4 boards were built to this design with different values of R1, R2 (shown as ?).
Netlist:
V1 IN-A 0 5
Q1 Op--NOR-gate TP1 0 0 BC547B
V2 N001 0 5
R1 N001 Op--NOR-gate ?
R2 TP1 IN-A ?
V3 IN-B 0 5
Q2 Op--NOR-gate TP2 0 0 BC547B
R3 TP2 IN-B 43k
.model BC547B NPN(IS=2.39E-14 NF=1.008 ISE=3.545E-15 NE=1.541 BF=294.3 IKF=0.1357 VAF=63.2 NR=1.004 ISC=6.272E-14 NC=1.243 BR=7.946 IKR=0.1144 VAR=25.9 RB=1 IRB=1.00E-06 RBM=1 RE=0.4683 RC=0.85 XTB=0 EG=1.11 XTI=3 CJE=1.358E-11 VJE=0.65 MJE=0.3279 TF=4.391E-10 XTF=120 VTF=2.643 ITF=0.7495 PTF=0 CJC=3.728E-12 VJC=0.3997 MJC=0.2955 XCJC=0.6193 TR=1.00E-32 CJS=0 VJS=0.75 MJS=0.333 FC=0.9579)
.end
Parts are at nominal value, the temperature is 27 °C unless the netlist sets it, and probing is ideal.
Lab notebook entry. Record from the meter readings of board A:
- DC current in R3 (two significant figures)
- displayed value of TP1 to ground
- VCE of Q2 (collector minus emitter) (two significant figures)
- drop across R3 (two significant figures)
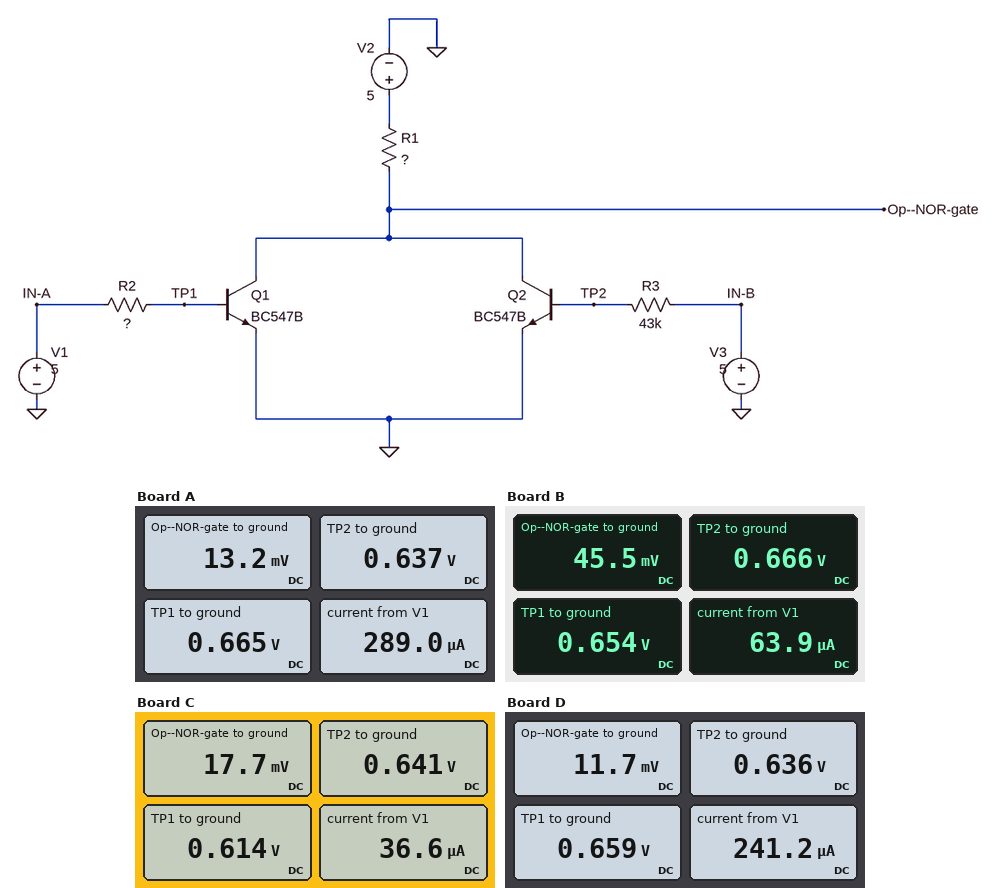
100 µA
0.665 V
13 mV
4.4 V
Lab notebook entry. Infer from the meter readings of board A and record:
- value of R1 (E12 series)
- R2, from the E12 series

6.8 kΩ
15 kΩ
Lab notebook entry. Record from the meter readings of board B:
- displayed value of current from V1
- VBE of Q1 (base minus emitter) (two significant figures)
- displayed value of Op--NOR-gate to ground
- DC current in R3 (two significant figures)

63.9 µA
650 mV
45.5 mV
100 µA
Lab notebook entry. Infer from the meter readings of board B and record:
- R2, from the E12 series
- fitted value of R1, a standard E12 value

68 kΩ
1.5 kΩ
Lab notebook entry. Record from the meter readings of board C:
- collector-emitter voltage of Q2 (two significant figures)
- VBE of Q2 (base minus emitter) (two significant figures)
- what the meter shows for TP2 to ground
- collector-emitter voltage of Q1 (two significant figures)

18 mV
640 mV
0.641 V
18 mV
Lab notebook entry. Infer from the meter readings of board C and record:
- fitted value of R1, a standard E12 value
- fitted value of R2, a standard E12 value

10 kΩ
120 kΩ
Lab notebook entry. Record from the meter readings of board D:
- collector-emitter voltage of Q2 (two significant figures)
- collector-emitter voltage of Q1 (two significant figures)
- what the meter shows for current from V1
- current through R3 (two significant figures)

12 mV
12 mV
241.2 µA
100 µA
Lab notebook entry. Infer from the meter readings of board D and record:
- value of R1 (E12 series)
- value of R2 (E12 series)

10 kΩ
18 kΩ
